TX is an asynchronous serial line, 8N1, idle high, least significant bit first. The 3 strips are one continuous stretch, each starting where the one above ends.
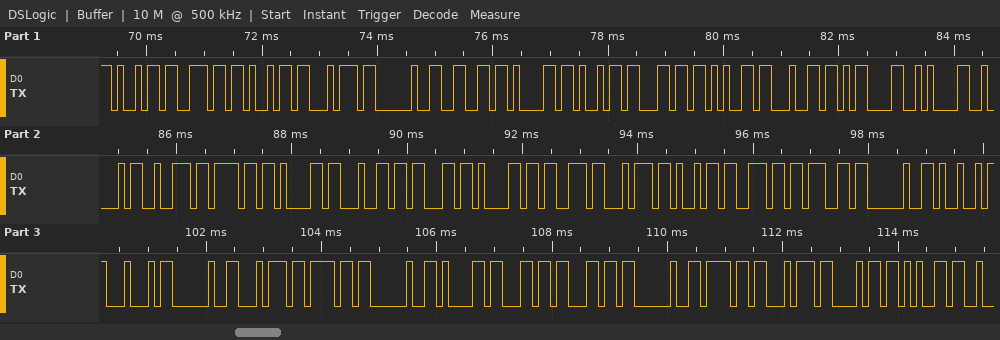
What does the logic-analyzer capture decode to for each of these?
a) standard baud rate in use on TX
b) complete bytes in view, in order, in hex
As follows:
9600 baud
69 6E 69 74 20 66 61 69 6C 65 64 0D 0A 42 72 6F 61 64 63 61 73 74 69 6E 67 20 49 44 20 74 6F 20 61 6C 6C 20 6F 74 68 65
